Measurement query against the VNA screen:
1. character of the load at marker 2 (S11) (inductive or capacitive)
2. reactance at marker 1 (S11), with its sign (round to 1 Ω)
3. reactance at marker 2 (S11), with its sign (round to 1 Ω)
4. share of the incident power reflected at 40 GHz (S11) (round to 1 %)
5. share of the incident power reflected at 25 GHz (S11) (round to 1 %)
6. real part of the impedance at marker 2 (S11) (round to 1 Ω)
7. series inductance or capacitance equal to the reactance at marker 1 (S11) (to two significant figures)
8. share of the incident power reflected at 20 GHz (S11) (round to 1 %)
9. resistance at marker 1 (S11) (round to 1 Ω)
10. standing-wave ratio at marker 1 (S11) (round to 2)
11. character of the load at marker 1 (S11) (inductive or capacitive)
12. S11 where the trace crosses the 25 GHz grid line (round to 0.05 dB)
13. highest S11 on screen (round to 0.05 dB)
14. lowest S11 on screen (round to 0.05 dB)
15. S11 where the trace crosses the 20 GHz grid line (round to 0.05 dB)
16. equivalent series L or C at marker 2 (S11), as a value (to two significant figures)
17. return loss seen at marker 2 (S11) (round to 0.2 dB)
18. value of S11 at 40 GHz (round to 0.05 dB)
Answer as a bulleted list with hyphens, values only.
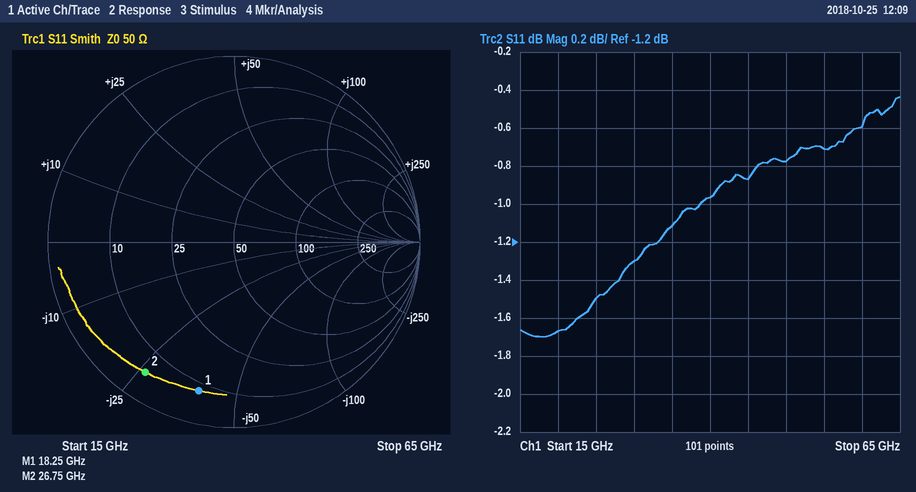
- capacitive
- -39 Ω
- -26 Ω
- 80 %
- 71 %
- 5 Ω
- 220 fF
- 68 %
- 8 Ω
- 10
- capacitive
- -1.50 dB
- -0.45 dB
- -1.70 dB
- -1.65 dB
- 230 fF
- 1.4 dB
- -0.95 dB
